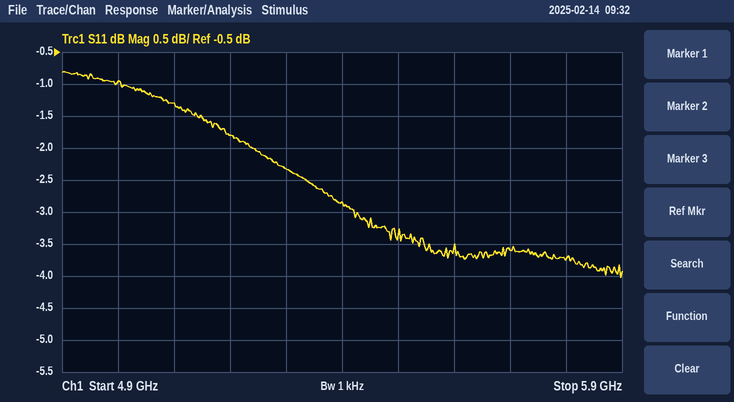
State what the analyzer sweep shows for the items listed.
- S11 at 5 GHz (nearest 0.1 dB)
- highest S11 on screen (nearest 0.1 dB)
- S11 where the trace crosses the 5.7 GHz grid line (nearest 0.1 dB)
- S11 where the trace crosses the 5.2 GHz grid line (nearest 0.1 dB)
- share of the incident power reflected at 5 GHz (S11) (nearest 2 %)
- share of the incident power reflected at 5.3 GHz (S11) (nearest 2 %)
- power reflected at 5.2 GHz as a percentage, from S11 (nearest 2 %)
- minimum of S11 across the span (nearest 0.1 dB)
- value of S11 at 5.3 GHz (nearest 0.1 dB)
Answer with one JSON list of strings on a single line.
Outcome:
["-1.0 dB", "-0.8 dB", "-3.6 dB", "-1.8 dB", "80 %", "58 %", "66 %", "-4.0 dB", "-2.3 dB"]
